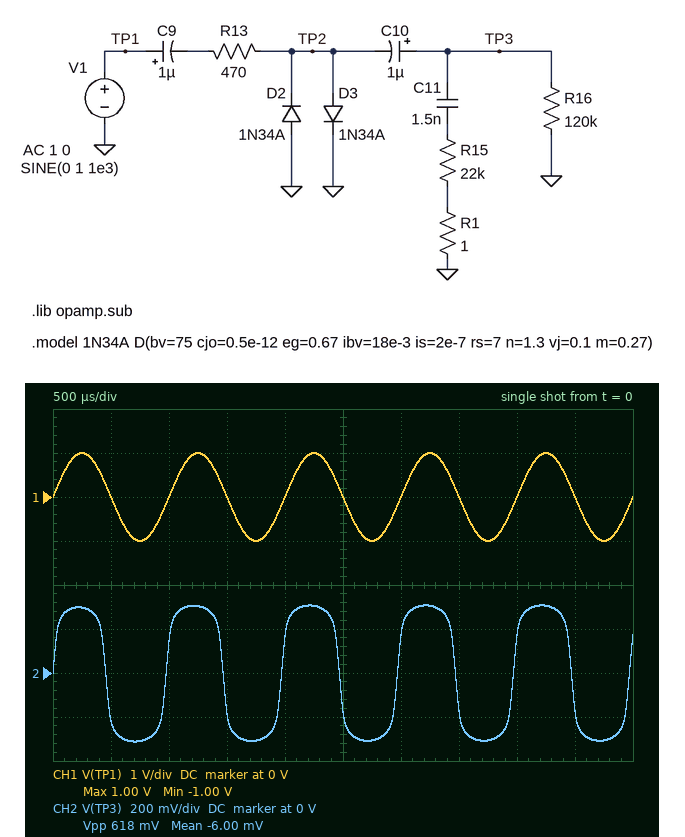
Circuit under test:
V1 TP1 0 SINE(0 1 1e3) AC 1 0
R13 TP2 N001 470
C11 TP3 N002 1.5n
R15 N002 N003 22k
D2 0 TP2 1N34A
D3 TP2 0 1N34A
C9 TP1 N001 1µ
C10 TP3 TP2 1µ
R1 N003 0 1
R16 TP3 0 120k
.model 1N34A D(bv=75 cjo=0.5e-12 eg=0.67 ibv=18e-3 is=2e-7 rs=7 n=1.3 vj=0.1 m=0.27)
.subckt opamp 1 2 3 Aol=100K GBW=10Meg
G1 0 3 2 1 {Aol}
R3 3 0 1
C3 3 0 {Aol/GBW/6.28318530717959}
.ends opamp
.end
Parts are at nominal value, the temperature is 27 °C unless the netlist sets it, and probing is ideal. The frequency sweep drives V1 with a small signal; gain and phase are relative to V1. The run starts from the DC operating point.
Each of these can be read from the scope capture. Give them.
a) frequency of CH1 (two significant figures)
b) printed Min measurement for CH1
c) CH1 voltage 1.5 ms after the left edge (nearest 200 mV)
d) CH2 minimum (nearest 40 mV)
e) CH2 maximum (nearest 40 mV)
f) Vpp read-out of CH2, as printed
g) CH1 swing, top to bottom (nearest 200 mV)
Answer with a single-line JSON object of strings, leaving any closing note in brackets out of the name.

{"frequency of CH1": "1.0 kHz", "printed Min measurement for CH1": "-1.00 V", "CH1 voltage 1.5 ms after the left edge": "0 V", "CH2 minimum": "-320 mV", "CH2 maximum": "320 mV", "Vpp read-out of CH2, as printed": "618 mV", "CH1 swing, top to bottom": "2.0 V"}
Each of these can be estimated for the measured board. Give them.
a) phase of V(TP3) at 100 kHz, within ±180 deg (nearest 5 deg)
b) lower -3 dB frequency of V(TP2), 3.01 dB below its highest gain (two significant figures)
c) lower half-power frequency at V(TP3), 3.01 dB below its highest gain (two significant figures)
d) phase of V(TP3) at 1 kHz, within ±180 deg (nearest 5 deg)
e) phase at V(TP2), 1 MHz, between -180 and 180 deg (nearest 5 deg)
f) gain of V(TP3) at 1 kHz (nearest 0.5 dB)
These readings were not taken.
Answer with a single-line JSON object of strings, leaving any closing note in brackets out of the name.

{"phase of V(TP3) at 100 kHz, within ±180 deg": "0 deg", "lower -3 dB frequency of V(TP2), 3.01 dB below its highest gain": "3.5 Hz", "lower half-power frequency at V(TP3), 3.01 dB below its highest gain": "4.0 Hz", "phase of V(TP3) at 1 kHz, within ±180 deg": "0 deg", "phase at V(TP2), 1 MHz, between -180 and 180 deg": "0 deg", "gain of V(TP3) at 1 kHz": "0 dB"}
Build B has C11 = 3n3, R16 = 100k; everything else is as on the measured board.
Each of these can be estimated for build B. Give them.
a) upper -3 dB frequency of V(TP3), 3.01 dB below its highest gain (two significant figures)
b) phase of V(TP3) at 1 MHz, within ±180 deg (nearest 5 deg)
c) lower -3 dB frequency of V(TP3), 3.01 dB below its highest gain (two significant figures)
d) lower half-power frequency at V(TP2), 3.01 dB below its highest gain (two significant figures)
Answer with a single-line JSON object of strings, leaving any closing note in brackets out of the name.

{"upper -3 dB frequency of V(TP3), 3.01 dB below its highest gain": "340 MHz", "phase of V(TP3) at 1 MHz, within ±180 deg": "0 deg", "lower -3 dB frequency of V(TP3), 3.01 dB below its highest gain": "4.4 Hz", "lower half-power frequency at V(TP2), 3.01 dB below its highest gain": "3.8 Hz"}
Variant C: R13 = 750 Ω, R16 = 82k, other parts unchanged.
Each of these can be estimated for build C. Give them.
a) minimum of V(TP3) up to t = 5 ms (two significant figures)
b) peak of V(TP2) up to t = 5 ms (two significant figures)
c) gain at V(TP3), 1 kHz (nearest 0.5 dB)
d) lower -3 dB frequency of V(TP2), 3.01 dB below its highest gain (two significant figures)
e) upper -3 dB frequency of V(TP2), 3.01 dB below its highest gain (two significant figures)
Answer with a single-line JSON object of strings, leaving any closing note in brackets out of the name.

{"minimum of V(TP3) up to t = 5 ms": "-290 mV", "peak of V(TP2) up to t = 5 ms": "290 mV", "gain at V(TP3), 1 kHz": "0 dB", "lower -3 dB frequency of V(TP2), 3.01 dB below its highest gain": "4.3 Hz", "upper -3 dB frequency of V(TP2), 3.01 dB below its highest gain": "210 MHz"}
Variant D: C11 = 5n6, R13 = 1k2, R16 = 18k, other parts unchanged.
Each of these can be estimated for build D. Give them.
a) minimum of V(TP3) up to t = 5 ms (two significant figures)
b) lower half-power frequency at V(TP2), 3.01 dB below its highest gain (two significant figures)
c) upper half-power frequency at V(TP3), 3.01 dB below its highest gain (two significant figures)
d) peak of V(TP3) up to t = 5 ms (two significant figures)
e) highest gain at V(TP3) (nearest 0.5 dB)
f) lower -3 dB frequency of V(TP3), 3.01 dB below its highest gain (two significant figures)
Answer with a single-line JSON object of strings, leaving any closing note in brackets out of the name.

{"minimum of V(TP3) up to t = 5 ms": "-280 mV", "lower half-power frequency at V(TP2), 3.01 dB below its highest gain": "12 Hz", "upper half-power frequency at V(TP3), 3.01 dB below its highest gain": "140 MHz", "peak of V(TP3) up to t = 5 ms": "270 mV", "highest gain at V(TP3)": "-1.0 dB", "lower -3 dB frequency of V(TP3), 3.01 dB below its highest gain": "17 Hz"}
